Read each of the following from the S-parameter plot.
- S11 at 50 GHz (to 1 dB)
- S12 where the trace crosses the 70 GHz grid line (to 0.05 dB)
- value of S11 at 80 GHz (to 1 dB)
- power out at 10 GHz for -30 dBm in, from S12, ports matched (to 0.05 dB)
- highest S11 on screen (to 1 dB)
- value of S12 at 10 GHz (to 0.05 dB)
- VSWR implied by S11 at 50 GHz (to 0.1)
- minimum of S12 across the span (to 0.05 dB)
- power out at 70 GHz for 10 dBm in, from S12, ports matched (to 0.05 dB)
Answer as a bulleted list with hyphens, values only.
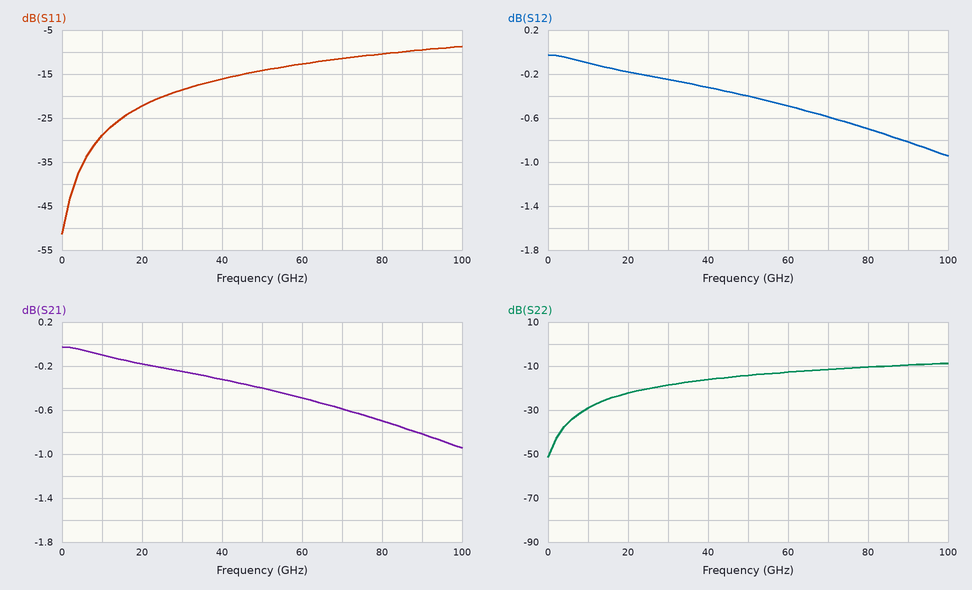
- -14 dB
- -0.60 dB
- -10 dB
- -30.10 dBm
- -9 dB
- -0.10 dB
- 1.5
- -0.95 dB
- 9.40 dBm
